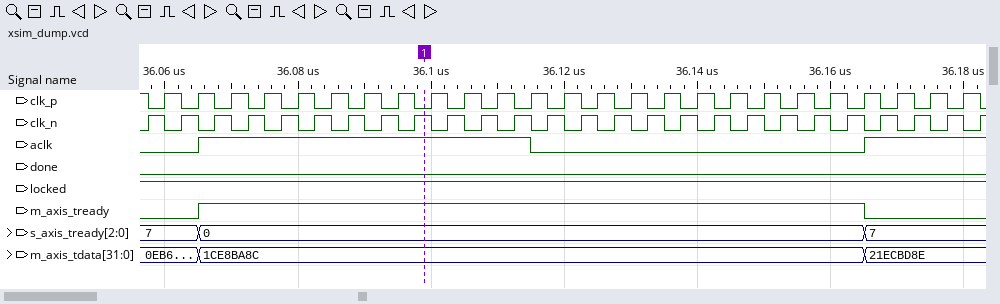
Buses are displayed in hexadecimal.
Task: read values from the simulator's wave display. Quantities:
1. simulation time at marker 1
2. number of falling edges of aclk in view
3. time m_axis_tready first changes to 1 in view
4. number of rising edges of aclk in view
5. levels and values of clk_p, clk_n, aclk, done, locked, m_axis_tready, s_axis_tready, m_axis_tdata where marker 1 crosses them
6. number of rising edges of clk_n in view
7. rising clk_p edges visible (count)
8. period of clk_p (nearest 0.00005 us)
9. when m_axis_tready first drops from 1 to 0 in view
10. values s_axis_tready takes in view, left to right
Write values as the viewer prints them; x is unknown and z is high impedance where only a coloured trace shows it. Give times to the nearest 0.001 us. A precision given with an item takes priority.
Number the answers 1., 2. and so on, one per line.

1. 36.099 us
2. 1
3. 36.065 us
4. 2
5. clk_p=0, clk_n=1, aclk=1, done=0, locked=1, m_axis_tready=1, s_axis_tready=0, m_axis_tdata=1CE8BA8C
6. 26
7. 25
8. 0.005 us
9. 36.165 us
10. 7, 0, 7
